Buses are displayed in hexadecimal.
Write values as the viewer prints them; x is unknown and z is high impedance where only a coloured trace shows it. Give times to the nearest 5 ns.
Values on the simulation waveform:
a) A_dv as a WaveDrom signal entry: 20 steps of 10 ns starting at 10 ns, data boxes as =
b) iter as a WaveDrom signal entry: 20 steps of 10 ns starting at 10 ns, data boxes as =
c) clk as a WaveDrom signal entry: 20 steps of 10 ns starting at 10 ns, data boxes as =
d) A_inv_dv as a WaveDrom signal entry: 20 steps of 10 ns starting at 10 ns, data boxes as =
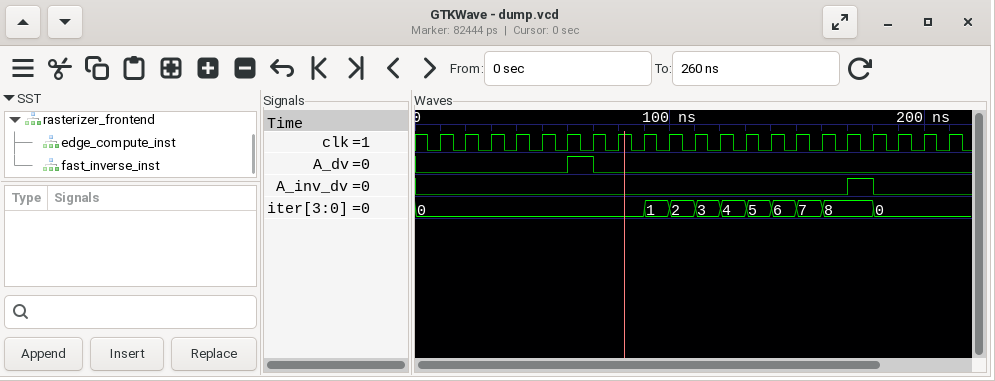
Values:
{name: 'A_dv', wave: '0....10.............'}
{name: 'iter', wave: '=.......========.=..', data: '0 1 2 3 4 5 6 7 8 0'}
{name: 'clk', wave: 'p...................'}
{name: 'A_inv_dv', wave: '0...............10..'}
